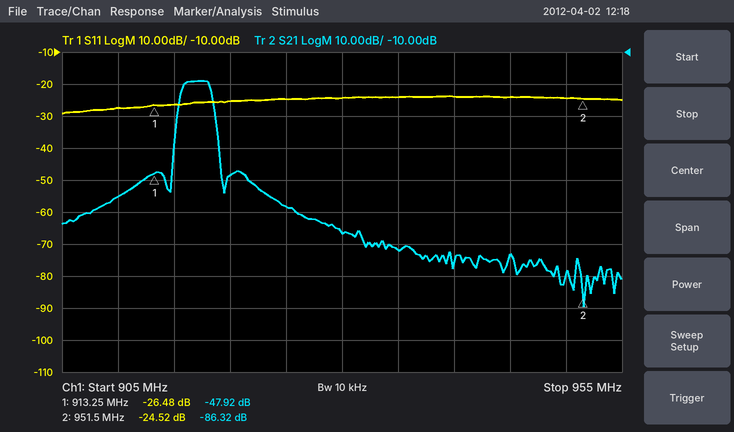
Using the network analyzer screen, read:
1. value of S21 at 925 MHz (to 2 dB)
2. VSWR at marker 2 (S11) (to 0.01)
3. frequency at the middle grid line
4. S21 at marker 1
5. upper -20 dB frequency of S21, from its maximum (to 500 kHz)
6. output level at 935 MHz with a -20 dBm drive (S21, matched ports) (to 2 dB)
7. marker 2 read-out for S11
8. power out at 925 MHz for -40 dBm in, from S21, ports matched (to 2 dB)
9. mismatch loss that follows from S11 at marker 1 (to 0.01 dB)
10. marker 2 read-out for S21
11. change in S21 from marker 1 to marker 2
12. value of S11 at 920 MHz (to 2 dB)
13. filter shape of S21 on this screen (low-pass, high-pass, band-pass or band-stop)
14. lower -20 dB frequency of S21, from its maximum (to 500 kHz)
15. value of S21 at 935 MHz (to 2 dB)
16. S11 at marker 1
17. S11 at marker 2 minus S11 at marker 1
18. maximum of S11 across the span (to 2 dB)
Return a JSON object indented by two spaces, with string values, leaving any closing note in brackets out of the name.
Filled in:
{
  "value of S21 at 925 MHz": "-58 dB",
  "VSWR at marker 2 (S11)": "1.13",
  "frequency at the middle grid line": "930 MHz",
  "S21 at marker 1": "-47.92 dB",
  "upper -20 dB frequency of S21, from its maximum": "919.0 MHz",
  "output level at 935 MHz with a -20 dBm drive (S21, matched ports)": "-92 dBm",
  "marker 2 read-out for S11": "-24.52 dB",
  "power out at 925 MHz for -40 dBm in, from S21, ports matched": "-98 dBm",
  "mismatch loss that follows from S11 at marker 1": "0.01 dB",
  "marker 2 read-out for S21": "-86.32 dB",
  "change in S21 from marker 1 to marker 2": "-38.40 dB",
  "value of S11 at 920 MHz": "-26 dB",
  "filter shape of S21 on this screen": "band-pass",
  "lower -20 dB frequency of S21, from its maximum": "915.0 MHz",
  "value of S21 at 935 MHz": "-72 dB",
  "S11 at marker 1": "-26.48 dB",
  "S11 at marker 2 minus S11 at marker 1": "1.96 dB",
  "maximum of S11 across the span": "-24 dB"
}
